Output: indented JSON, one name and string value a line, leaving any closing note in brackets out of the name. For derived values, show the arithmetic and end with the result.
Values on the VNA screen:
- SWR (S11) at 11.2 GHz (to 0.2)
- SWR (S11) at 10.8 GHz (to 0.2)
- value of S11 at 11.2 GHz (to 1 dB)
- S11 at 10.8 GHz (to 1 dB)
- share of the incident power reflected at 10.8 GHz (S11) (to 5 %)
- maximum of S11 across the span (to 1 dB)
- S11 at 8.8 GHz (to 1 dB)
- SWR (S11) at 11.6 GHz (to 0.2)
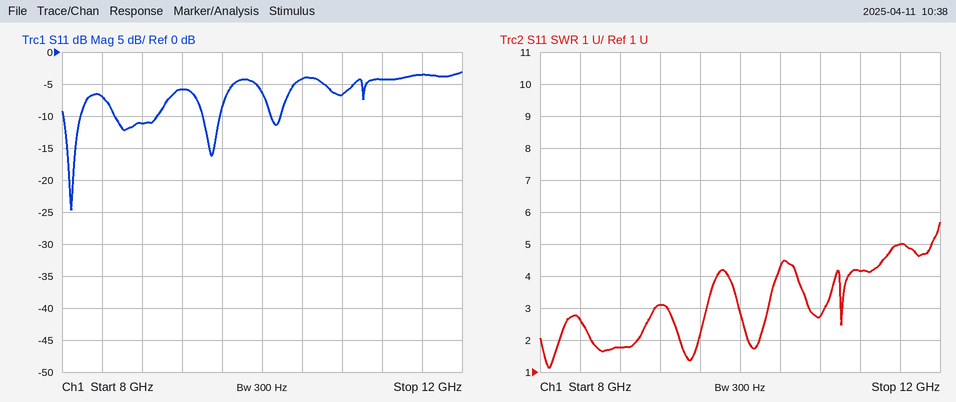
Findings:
{
  "SWR (S11) at 11.2 GHz": "4.2",
  "SWR (S11) at 10.8 GHz": "2.8",
  "value of S11 at 11.2 GHz": "-4 dB",
  "S11 at 10.8 GHz": "-7 dB",
  "share of the incident power reflected at 10.8 GHz (S11)": "10^(-7/10) ≈ 20 %",
  "maximum of S11 across the span": "-3 dB",
  "S11 at 8.8 GHz": "-11 dB",
  "SWR (S11) at 11.6 GHz": "5.0"
}
